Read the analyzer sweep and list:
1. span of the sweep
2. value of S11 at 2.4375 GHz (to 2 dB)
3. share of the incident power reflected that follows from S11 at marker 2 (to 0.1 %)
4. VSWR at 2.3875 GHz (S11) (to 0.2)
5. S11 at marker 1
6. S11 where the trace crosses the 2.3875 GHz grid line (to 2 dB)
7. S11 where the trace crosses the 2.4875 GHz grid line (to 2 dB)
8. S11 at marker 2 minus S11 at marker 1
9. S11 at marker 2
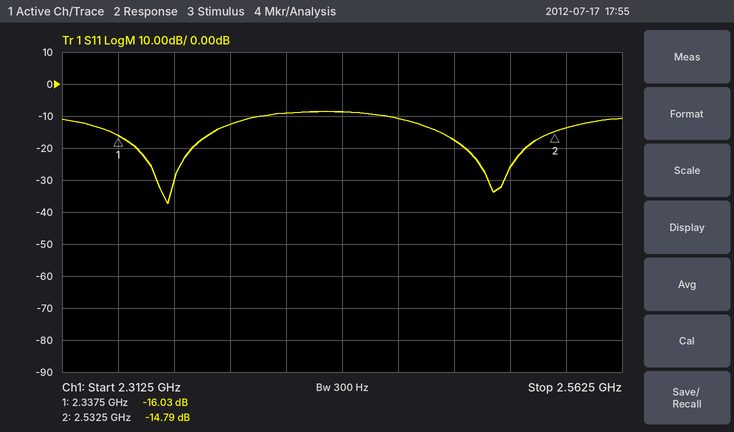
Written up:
250 MHz
-8 dB
3.3 %
1.6
-16.03 dB
-12 dB
-18 dB
1.24 dB
-14.79 dB
